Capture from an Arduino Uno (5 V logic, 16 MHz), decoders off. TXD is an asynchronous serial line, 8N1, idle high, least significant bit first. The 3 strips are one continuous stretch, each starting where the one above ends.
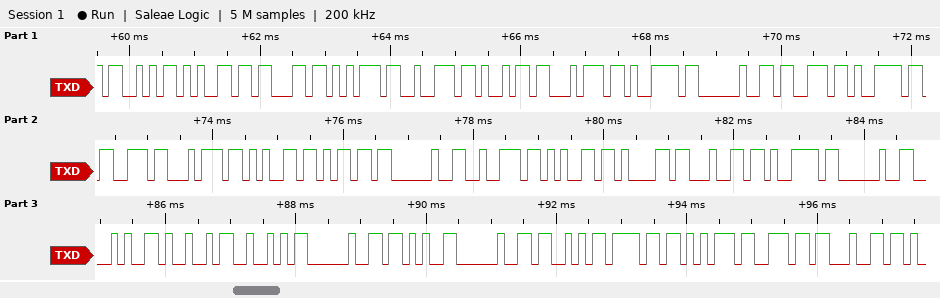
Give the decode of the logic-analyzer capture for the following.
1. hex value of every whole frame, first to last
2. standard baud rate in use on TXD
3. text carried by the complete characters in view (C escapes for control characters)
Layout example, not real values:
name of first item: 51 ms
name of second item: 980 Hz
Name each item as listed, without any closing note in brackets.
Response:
hex value of every whole frame, first to last: 53 65 63 75 72 69 74 79 20 73 79 73 74 65 6D 20 72 65 61 64 79 20 28 49 52 20 2B 20 53 6F 75 6E 64
standard baud rate in use on TXD: 9600 baud
text carried by the complete characters in view: "Security system ready (IR + Sound"
